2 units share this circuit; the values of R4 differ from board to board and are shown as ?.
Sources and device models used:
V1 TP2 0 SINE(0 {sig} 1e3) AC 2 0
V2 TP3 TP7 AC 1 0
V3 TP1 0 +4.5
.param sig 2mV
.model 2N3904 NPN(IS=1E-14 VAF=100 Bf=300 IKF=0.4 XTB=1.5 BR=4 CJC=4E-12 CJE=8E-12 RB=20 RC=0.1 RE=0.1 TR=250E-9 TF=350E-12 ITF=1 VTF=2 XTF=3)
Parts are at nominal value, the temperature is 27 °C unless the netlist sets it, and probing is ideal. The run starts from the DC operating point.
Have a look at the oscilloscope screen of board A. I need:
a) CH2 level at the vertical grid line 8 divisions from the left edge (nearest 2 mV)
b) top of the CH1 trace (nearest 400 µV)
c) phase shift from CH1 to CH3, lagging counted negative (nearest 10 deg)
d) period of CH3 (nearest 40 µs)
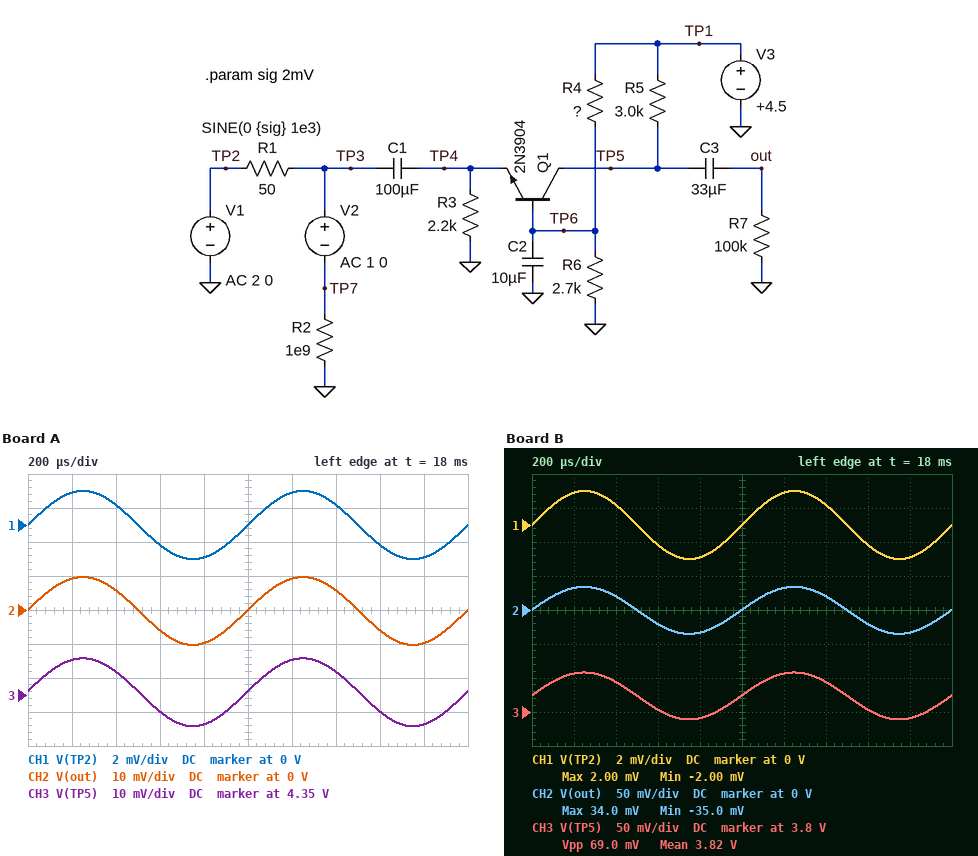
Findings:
-6 mV
2.0 mV
0 deg
1.00 ms
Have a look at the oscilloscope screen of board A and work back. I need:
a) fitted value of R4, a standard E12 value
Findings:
15 kΩ
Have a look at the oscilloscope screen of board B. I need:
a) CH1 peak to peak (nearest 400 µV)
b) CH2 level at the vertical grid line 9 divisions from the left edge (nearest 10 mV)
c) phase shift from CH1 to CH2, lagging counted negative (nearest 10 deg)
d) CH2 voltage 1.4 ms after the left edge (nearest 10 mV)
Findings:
4.0 mV
-30 mV
0 deg
20 mV
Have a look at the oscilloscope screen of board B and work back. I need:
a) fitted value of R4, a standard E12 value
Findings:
8.2 kΩ
